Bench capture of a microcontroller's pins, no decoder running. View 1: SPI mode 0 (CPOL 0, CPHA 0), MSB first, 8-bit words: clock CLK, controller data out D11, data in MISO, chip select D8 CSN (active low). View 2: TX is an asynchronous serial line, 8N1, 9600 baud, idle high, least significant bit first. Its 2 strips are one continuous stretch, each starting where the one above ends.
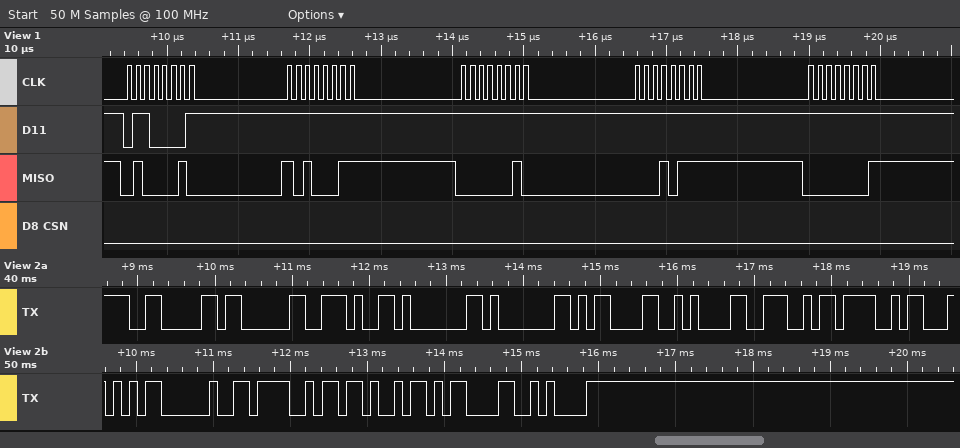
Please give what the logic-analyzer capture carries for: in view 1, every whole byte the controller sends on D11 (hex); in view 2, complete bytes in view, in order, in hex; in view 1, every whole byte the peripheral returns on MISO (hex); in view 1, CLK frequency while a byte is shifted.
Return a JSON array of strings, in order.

["0x61 0xFF 0xFF 0xFF 0xFF", "06 03 2E 01 01 0D 0A 4E 4F 54 20 4F 4B 0D 0A", "0x42 0xA3 0x02 0x17 0x01", "8 MHz"]
